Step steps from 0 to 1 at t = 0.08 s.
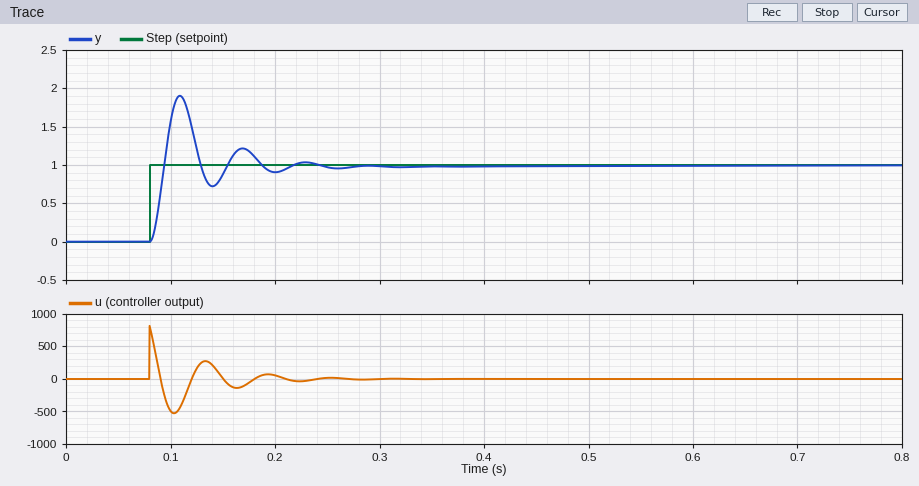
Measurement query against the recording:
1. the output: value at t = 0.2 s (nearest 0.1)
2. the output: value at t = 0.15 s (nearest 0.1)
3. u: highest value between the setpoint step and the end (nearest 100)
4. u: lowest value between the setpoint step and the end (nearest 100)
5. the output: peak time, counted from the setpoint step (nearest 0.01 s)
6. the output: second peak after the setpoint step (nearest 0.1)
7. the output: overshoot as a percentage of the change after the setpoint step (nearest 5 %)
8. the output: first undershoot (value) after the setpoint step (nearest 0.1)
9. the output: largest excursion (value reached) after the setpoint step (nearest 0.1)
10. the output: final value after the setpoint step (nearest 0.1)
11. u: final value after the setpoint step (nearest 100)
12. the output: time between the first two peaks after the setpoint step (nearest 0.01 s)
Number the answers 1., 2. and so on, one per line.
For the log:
1. 0.9
2. 0.9
3. 800
4. -500
5. 0.03 s
6. 1.2
7. 90 %
8. 0.7
9. 1.9
10. 1.0
11. 0
12. 0.06 s
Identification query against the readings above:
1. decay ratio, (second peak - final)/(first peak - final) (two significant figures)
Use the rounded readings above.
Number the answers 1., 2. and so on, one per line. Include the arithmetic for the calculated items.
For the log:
1. (1.2 - 1) / (1.9 - 1) = 0.22
